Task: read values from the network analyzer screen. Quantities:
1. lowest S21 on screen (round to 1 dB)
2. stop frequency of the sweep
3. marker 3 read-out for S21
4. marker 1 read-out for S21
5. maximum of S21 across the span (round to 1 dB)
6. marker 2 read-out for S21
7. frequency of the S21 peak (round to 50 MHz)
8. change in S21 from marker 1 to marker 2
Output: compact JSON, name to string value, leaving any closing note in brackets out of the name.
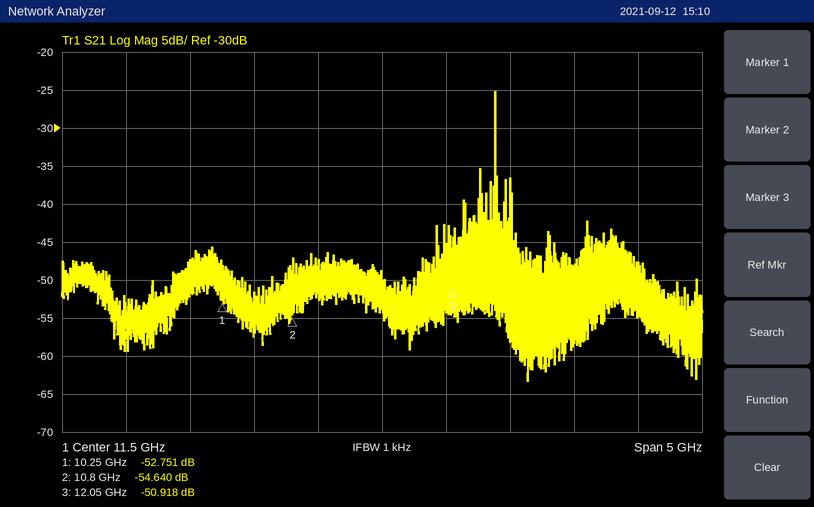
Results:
{"lowest S21 on screen": "-63 dB", "stop frequency of the sweep": "14 GHz", "marker 3 read-out for S21": "-50.918 dB", "marker 1 read-out for S21": "-52.751 dB", "maximum of S21 across the span": "-25 dB", "marker 2 read-out for S21": "-54.640 dB", "frequency of the S21 peak": "12.40 GHz", "change in S21 from marker 1 to marker 2": "-1.889 dB"}
